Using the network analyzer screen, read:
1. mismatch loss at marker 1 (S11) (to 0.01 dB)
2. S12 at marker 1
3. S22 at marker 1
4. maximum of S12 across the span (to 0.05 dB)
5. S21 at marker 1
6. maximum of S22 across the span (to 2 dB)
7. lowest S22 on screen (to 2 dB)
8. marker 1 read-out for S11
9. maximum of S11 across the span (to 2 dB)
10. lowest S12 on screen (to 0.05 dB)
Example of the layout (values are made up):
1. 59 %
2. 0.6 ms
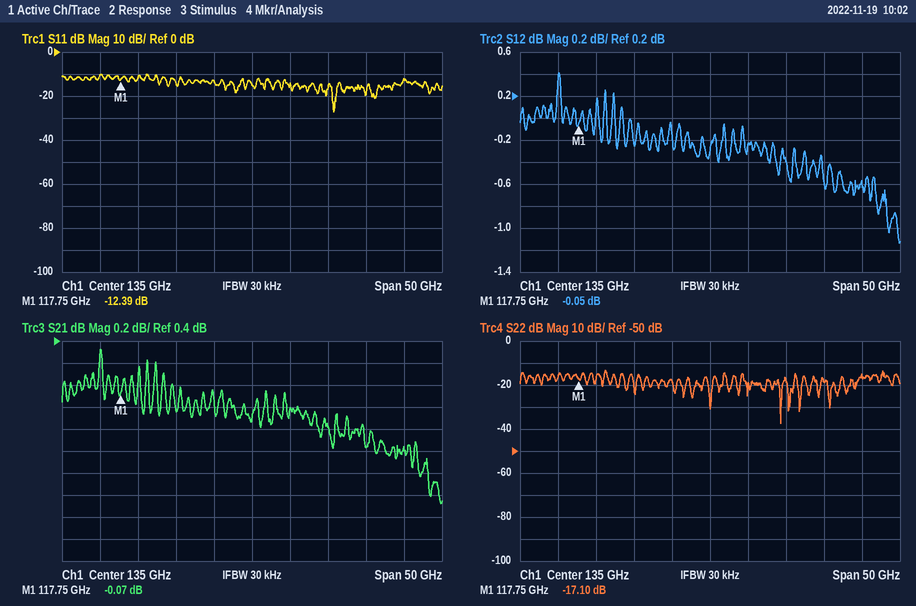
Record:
1. 0.26 dB
2. -0.05 dB
3. -17.10 dB
4. 0.40 dB
5. -0.07 dB
6. -14 dB
7. -38 dB
8. -12.39 dB
9. -10 dB
10. -1.15 dB
